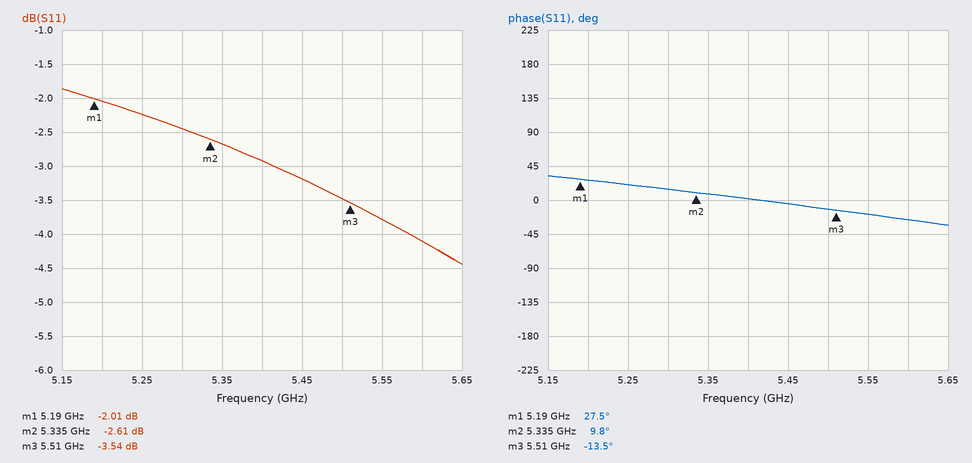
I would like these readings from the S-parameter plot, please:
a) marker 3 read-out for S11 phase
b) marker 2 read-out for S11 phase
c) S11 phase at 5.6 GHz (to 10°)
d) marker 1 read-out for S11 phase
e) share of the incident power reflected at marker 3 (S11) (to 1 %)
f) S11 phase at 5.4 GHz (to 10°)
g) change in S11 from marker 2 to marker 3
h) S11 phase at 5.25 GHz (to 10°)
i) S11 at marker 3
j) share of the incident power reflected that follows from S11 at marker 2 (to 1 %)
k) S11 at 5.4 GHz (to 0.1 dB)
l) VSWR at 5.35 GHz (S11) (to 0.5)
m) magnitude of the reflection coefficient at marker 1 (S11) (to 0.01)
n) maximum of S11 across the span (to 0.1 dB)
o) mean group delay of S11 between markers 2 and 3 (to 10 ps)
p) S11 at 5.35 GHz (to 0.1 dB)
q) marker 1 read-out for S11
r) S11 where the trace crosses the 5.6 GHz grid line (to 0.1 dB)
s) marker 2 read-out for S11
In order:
-13.5°
9.8°
-30°
27.5°
44 %
0°
-0.93 dB
20°
-3.54 dB
55 %
-2.9 dB
6.5
0.79
-1.9 dB
370 ps
-2.7 dB
-2.01 dB
-4.1 dB
-2.61 dB
